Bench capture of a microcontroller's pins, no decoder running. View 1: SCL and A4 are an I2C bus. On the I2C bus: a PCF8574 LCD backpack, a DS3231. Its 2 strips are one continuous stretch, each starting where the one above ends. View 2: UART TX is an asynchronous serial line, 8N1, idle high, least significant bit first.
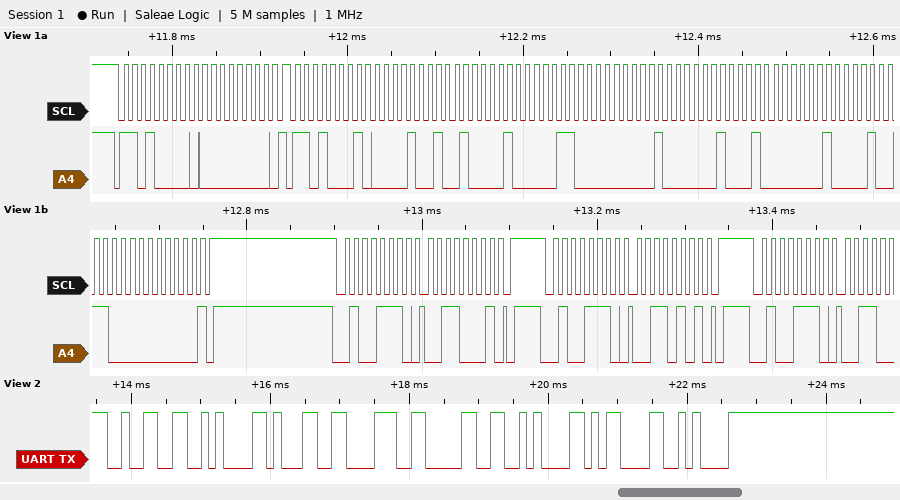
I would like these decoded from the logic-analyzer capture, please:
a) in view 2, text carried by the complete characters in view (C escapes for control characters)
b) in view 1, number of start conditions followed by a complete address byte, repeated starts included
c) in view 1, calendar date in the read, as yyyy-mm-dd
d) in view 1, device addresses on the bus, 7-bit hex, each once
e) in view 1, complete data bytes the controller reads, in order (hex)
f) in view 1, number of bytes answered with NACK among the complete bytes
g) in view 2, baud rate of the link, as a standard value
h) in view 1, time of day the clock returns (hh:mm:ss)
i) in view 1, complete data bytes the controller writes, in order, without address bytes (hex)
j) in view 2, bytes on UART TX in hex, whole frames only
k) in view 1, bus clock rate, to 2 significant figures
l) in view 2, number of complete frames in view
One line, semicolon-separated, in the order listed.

"2\n180\n\r\n"; 5; 2026-02-11; 0x68 0x27; 09 42 18 04 11 02 26 00; 1; 9600 baud; 18:42:09; 00 31 35; 0x32 0x0A 0x31 0x38 0x30 0x0A 0x0D 0x0A; 100 kHz; 8
